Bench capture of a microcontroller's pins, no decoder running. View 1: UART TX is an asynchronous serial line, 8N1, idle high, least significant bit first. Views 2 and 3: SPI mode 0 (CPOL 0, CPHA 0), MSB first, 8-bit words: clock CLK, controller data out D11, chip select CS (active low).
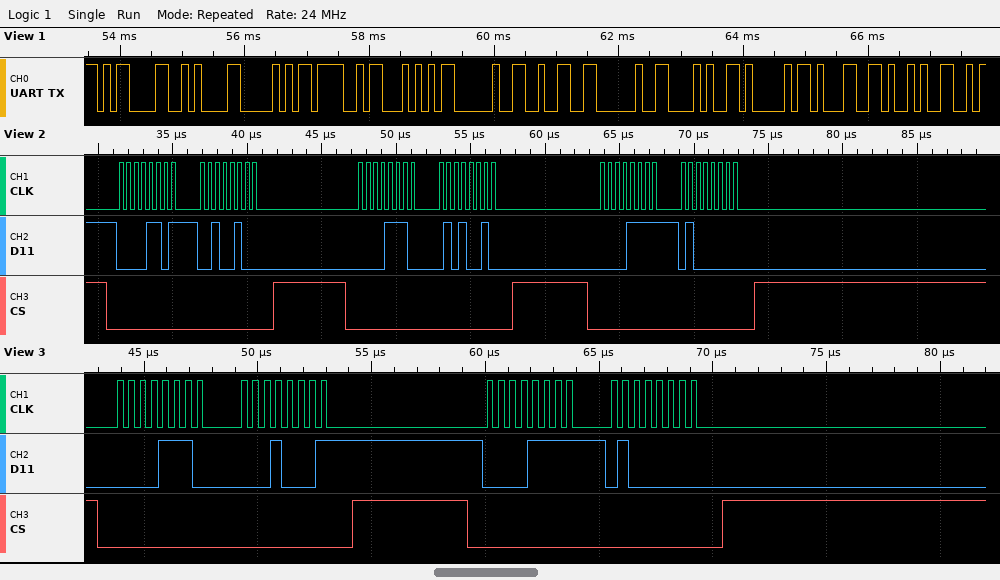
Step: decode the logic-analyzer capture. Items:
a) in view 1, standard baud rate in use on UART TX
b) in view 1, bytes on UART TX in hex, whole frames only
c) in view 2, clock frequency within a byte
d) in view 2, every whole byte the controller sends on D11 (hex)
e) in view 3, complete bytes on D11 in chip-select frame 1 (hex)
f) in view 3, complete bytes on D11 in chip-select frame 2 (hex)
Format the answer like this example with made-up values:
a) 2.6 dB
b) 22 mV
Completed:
a) 9600 baud
b) 0D 0A 50 4F 54 20 32 20 28 41 31 29
c) 2 MHz
d) 0D 24 0E 52 0F 40
e) 0E 11
f) 0F 40
